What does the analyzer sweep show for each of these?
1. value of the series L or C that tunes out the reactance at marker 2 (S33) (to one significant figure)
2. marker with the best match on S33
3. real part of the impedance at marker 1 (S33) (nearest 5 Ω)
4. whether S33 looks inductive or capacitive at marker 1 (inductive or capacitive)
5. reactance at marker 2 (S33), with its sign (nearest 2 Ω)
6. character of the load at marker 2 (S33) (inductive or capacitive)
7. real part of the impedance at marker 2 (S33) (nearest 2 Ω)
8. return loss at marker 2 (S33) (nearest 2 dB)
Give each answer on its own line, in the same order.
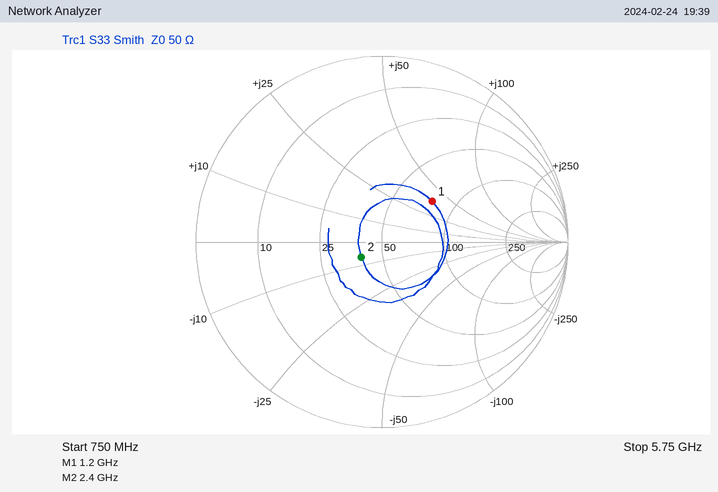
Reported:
400 pH
marker 2
75 Ω
inductive
-6 Ω
capacitive
40 Ω
18 dB
